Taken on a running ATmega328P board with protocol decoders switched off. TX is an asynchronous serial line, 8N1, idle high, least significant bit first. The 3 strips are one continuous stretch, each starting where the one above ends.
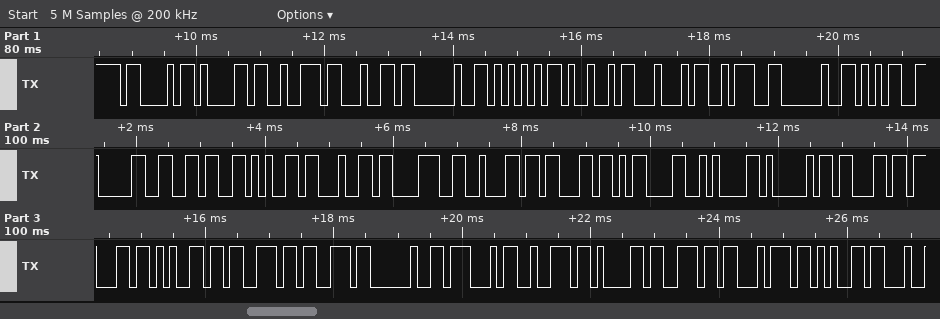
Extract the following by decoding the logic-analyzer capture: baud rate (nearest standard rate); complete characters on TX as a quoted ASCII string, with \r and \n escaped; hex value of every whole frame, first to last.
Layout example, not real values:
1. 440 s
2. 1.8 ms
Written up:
1. 9600 baud
2. "Card UID: 506ed8bc\r\nAccess Grante"
3. 43 61 72 64 20 55 49 44 3A 20 35 30 36 65 64 38 62 63 0D 0A 41 63 63 65 73 73 20 47 72 61 6E 74 65
